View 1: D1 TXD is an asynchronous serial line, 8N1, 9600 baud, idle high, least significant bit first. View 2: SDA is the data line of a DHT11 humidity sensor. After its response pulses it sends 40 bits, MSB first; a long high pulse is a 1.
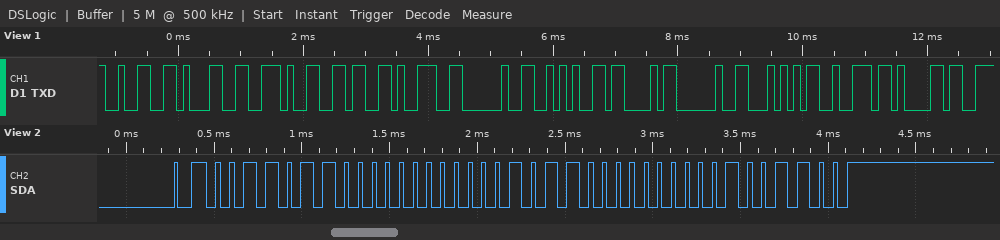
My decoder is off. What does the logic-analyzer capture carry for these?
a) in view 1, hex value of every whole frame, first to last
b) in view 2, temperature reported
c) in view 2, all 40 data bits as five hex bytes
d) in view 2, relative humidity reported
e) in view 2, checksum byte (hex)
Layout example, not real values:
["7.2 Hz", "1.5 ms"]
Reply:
["32 31 2E 36 39 20 2A 43 20 54 72 61", "22.0 °C", "36 00 16 00 4C", "54 %", "0x4C"]
